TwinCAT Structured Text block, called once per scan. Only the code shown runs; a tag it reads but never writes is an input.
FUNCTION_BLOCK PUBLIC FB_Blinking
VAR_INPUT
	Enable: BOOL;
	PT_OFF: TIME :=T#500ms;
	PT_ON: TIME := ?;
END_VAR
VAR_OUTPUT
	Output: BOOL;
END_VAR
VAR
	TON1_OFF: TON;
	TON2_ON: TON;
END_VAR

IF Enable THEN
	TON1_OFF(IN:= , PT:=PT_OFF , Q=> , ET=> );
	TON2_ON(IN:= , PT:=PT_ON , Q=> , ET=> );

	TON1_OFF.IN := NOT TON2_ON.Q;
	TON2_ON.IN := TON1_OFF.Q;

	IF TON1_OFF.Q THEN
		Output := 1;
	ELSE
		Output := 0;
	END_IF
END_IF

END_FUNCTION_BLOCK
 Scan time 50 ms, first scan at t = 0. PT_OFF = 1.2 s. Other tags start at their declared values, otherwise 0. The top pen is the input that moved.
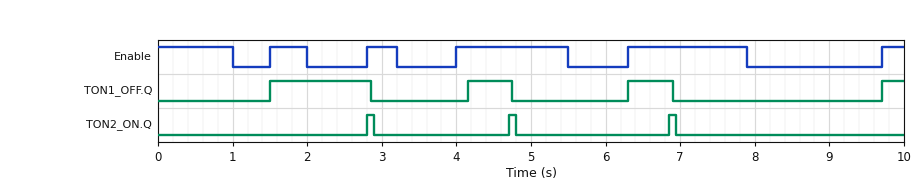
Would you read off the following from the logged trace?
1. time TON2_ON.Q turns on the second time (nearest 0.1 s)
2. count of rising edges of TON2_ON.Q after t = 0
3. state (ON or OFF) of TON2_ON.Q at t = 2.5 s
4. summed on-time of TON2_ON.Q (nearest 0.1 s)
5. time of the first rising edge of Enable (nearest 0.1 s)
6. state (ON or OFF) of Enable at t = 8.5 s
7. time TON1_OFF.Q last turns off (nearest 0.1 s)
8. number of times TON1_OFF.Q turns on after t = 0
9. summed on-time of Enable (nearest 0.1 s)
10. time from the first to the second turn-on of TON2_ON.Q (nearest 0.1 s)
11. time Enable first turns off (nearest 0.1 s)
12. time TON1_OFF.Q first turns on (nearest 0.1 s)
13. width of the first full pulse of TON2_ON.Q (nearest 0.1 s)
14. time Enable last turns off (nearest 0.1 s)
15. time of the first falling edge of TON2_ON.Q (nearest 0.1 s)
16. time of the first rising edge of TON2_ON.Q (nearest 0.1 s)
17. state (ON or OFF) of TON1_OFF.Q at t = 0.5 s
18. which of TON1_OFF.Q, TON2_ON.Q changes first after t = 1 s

4.7 s
3
OFF
0.3 s
1.5 s
OFF
6.9 s
4
5.3 s
1.9 s
1.0 s
1.5 s
0.1 s
7.9 s
2.9 s
2.8 s
OFF
TON1_OFF.Q
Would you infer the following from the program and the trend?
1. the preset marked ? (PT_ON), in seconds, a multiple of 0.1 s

0.5 s
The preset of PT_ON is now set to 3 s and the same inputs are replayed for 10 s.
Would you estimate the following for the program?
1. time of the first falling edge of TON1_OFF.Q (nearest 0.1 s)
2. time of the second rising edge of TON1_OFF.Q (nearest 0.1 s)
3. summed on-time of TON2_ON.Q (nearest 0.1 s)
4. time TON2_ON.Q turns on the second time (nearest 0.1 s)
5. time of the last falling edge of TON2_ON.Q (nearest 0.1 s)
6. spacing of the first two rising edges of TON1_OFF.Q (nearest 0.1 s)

4.6 s
6.3 s
0.2 s
9.7 s
9.8 s
4.8 s
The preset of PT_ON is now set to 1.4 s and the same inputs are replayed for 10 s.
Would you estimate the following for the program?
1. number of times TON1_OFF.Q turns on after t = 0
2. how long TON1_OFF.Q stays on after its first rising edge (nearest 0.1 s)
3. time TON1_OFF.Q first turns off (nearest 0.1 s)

3
1.5 s
3.0 s
